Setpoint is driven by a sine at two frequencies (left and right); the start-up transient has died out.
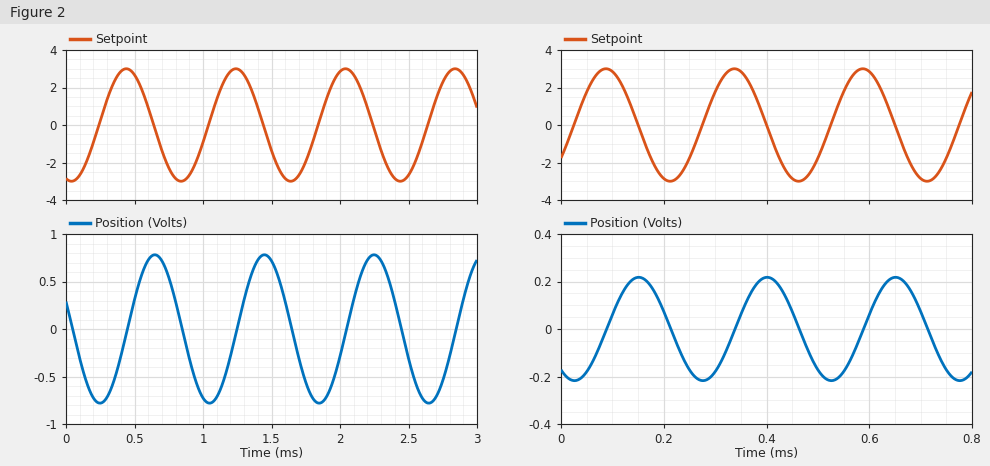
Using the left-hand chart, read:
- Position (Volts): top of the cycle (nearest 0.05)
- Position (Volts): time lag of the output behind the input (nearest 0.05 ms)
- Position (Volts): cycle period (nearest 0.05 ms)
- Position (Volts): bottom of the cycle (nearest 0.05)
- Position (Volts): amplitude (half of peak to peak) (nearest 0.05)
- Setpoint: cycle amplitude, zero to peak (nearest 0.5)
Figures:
0.80
0.20 ms
0.80 ms
-0.80
0.80
3.0
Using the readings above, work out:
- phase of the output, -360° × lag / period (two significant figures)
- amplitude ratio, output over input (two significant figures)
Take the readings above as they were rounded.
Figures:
-90°
0.27
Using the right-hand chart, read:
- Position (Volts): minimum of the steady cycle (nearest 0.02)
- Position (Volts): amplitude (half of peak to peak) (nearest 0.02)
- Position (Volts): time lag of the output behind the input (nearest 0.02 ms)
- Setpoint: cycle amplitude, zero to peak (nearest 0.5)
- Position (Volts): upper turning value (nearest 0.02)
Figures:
-0.22
0.22
0.06 ms
3.0
0.22
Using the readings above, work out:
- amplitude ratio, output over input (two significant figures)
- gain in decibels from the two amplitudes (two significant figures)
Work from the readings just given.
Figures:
0.073
-23 dB
